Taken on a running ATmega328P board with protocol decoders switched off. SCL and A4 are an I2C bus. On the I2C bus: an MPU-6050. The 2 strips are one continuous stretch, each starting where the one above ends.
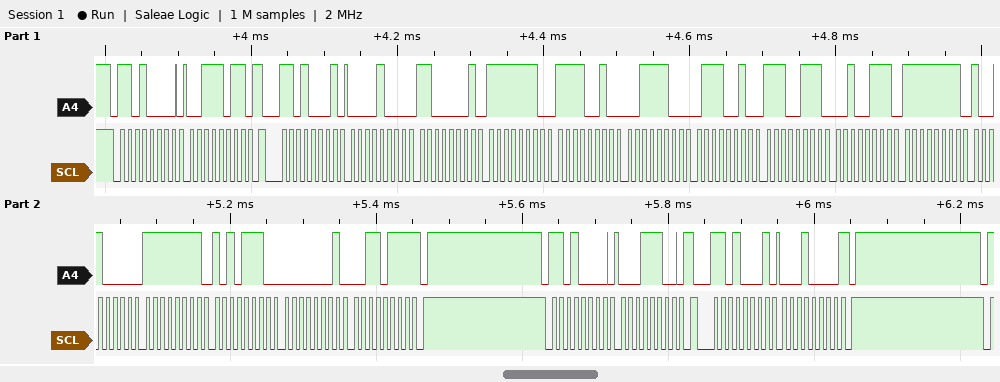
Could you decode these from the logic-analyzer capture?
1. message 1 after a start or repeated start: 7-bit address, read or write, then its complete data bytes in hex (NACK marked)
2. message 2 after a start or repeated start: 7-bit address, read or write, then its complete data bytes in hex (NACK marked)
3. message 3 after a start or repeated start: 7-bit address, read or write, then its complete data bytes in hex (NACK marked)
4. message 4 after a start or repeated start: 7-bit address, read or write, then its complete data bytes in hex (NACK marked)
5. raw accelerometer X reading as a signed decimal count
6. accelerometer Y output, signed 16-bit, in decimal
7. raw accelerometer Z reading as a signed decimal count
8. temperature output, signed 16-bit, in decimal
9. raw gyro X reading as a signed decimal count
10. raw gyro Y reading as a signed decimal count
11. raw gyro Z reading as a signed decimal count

0x68 write: 3B
0x68 read: 08 C1 FE F2 3C 72 E7 27 FF 90 FF AE 01 37 NACK
0x68 write: 1C
0x68 read: 10 NACK
2241
-270
15474
-6361
-112
-82
311
